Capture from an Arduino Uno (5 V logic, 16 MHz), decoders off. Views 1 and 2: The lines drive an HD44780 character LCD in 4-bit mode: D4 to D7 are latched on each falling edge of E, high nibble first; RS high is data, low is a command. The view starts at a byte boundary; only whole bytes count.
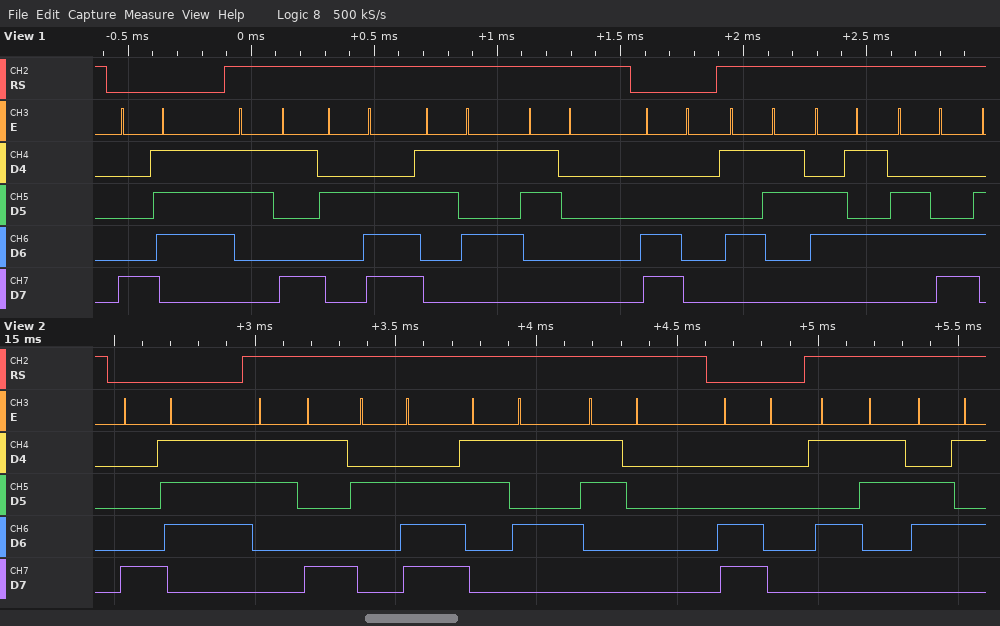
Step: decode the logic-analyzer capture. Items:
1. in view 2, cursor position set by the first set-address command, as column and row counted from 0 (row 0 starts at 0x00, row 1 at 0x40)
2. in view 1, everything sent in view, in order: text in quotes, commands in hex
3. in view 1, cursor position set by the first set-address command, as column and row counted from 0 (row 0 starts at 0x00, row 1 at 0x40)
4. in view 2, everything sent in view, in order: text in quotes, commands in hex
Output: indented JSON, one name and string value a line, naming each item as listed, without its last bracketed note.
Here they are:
{
  "in view 2, cursor position set by the first set-address command, as column and row counted from 0": "column 7, row 0",
  "in view 1, everything sent in view, in order: text in quotes, commands in hex": "0x87 \"9.50\" 0xC0 \"Sel\"",
  "in view 1, cursor position set by the first set-address command, as column and row counted from 0": "column 7, row 0",
  "in view 2, everything sent in view, in order: text in quotes, commands in hex": "0x87 \"9.50\" 0xC0 \"Se\""
}
